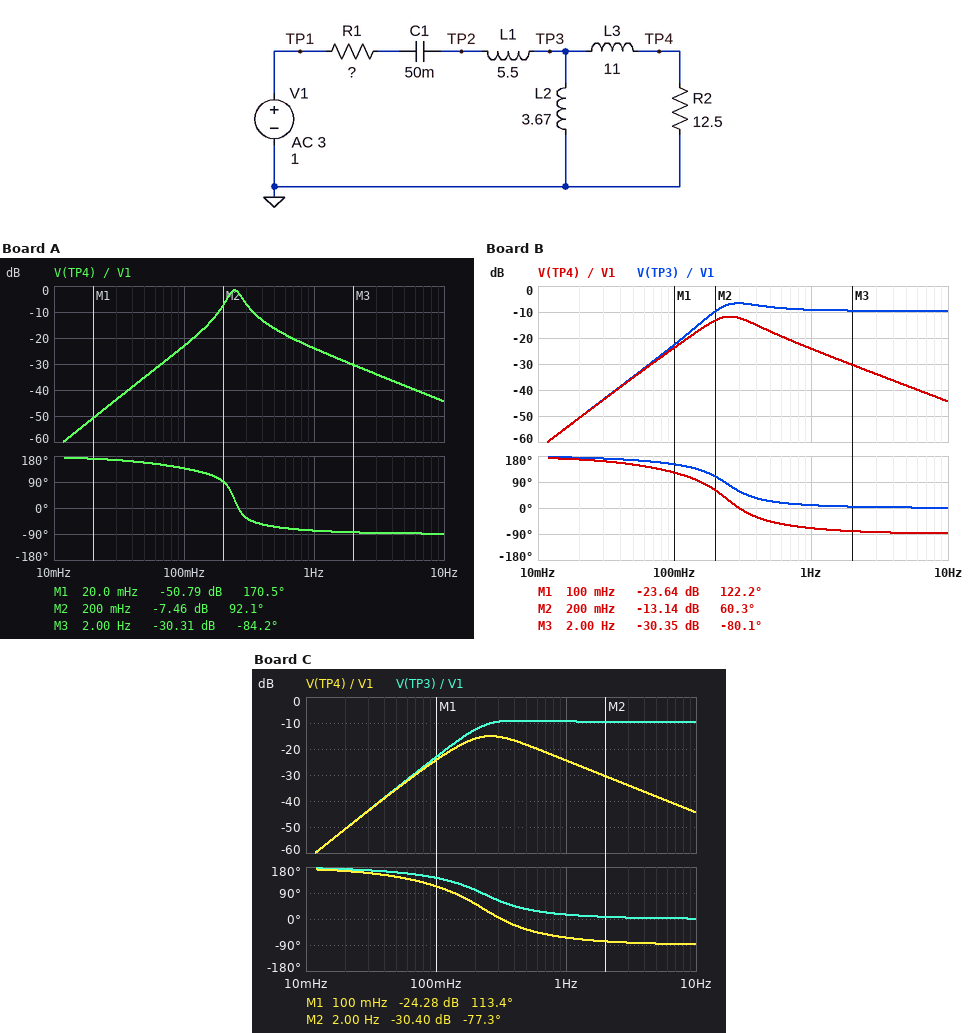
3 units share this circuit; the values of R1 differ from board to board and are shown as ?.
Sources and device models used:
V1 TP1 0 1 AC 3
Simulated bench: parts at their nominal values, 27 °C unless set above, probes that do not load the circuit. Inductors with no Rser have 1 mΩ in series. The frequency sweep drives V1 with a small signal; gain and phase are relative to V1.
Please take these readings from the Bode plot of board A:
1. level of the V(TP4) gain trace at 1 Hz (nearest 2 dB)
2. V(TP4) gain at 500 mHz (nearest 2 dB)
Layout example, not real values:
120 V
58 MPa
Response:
-24 dB
-16 dB
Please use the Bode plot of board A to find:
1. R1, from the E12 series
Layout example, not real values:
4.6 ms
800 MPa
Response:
2.7 Ω
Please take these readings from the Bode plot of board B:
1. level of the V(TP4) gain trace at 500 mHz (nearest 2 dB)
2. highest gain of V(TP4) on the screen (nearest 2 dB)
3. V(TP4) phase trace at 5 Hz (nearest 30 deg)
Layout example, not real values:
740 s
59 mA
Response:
-18 dB
-12 dB
-90 deg
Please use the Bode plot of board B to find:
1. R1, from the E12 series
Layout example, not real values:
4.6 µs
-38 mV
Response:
10 Ω
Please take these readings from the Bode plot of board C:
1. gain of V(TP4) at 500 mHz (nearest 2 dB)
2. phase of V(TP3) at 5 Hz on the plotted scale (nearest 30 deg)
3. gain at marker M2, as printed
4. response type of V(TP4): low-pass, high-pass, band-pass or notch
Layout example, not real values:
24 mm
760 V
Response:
-18 dB
0 deg
-30.40 dB
band-pass
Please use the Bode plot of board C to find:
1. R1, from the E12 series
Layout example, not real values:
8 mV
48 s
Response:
15 Ω
